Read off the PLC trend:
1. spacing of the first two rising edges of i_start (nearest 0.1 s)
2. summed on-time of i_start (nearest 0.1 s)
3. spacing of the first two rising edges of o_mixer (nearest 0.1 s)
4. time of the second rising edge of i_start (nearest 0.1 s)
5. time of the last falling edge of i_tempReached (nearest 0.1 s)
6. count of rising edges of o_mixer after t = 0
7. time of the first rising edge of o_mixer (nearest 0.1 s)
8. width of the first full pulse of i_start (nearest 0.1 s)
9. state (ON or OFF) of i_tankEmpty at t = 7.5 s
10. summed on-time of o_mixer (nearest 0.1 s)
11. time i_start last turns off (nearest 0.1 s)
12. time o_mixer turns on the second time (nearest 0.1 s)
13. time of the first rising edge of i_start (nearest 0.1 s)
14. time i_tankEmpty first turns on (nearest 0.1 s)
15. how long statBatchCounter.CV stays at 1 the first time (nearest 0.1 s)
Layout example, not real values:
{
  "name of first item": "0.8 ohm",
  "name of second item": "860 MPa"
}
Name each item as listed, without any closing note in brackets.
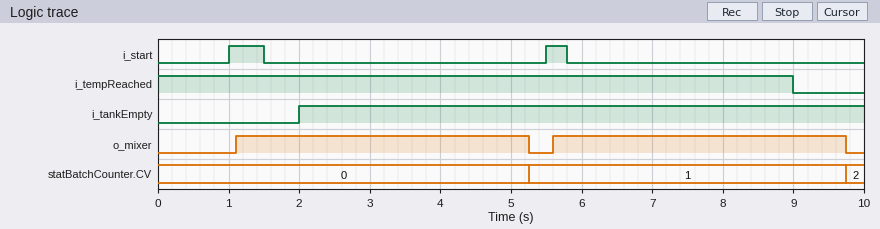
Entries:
{
  "spacing of the first two rising edges of i_start": "4.5 s",
  "summed on-time of i_start": "0.8 s",
  "spacing of the first two rising edges of o_mixer": "4.5 s",
  "time of the second rising edge of i_start": "5.5 s",
  "time of the last falling edge of i_tempReached": "9.0 s",
  "count of rising edges of o_mixer after t = 0": "2",
  "time of the first rising edge of o_mixer": "1.1 s",
  "width of the first full pulse of i_start": "0.5 s",
  "state (ON or OFF) of i_tankEmpty at t = 7.5 s": "ON",
  "summed on-time of o_mixer": "8.3 s",
  "time i_start last turns off": "5.8 s",
  "time o_mixer turns on the second time": "5.6 s",
  "time of the first rising edge of i_start": "1.0 s",
  "time i_tankEmpty first turns on": "2.0 s",
  "how long statBatchCounter.CV stays at 1 the first time": "4.5 s"
}
